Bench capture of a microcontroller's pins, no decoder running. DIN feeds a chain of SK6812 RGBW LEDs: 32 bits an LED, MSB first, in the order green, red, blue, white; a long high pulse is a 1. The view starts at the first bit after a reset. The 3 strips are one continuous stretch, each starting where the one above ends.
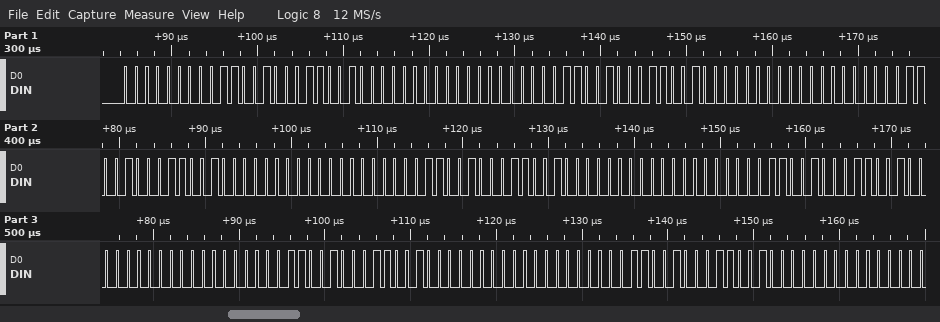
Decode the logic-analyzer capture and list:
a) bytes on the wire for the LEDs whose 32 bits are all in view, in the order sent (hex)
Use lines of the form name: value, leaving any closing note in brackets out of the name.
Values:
bytes on the wire for the LEDs whose 32 bits are all in view, in the order sent: 00 64 64 00 00 64 64 00 00 64 64 00 00 64 64 00 00 64 64 00 00 64 64 00 00 64 64 00
